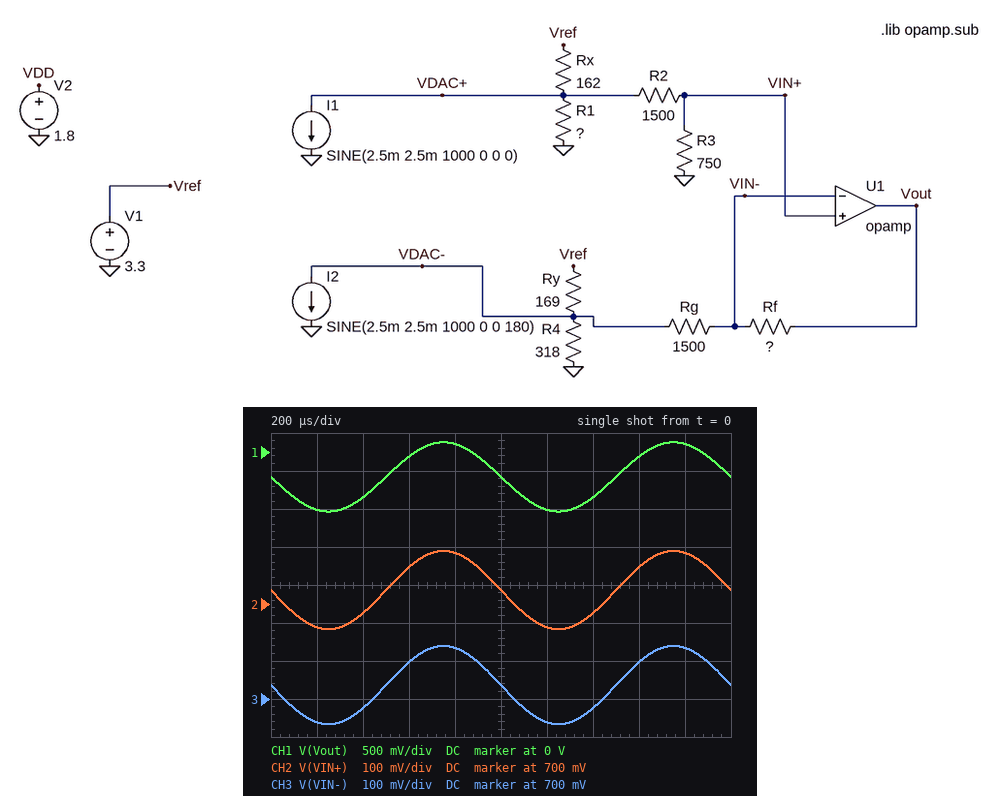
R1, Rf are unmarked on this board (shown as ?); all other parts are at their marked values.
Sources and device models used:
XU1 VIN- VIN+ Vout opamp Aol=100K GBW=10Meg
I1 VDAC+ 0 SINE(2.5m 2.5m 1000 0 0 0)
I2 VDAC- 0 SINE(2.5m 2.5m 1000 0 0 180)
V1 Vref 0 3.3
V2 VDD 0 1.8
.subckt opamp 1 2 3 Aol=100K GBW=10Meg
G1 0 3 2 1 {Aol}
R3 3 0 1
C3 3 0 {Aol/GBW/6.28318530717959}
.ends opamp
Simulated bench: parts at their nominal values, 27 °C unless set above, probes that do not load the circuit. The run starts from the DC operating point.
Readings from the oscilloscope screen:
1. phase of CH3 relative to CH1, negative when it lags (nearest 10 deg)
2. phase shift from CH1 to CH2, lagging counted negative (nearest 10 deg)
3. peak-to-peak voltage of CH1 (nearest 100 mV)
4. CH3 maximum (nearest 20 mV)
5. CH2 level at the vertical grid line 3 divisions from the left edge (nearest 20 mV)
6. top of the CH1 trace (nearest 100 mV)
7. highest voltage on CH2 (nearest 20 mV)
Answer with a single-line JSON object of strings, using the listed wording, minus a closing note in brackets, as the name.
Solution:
{"phase of CH3 relative to CH1, negative when it lags": "0 deg", "phase shift from CH1 to CH2, lagging counted negative": "0 deg", "peak-to-peak voltage of CH1": "900 mV", "CH3 maximum": "840 mV", "CH2 level at the vertical grid line 3 divisions from the left edge": "800 mV", "top of the CH1 trace": "100 mV", "highest voltage on CH2": "840 mV"}
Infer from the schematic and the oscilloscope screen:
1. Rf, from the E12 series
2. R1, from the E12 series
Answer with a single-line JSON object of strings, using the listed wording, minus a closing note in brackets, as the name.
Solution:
{"Rf, from the E12 series": "1.5 kΩ", "R1, from the E12 series": "680 Ω"}
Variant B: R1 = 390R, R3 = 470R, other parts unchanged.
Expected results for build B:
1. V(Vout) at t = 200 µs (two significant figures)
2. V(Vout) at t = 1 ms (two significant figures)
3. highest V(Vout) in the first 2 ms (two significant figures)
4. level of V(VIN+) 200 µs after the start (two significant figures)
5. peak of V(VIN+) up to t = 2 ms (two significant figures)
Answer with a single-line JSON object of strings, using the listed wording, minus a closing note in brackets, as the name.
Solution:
{"V(Vout) at t = 200 µs": "-1.2 V", "V(Vout) at t = 1 ms": "-860 mV", "highest V(Vout) in the first 2 ms": "-480 mV", "level of V(VIN+) 200 µs after the start": "400 mV", "peak of V(VIN+) up to t = 2 ms": "530 mV"}
